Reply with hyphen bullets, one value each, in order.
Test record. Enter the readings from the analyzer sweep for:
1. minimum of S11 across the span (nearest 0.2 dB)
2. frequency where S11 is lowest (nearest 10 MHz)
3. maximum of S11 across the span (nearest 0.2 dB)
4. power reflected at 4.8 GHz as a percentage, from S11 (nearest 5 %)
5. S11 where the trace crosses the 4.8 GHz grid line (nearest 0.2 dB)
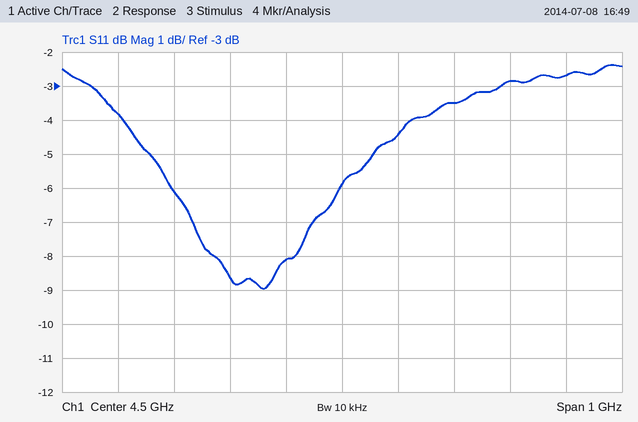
- -9.0 dB
- 4.36 GHz
- -2.4 dB
- 50 %
- -2.8 dB
